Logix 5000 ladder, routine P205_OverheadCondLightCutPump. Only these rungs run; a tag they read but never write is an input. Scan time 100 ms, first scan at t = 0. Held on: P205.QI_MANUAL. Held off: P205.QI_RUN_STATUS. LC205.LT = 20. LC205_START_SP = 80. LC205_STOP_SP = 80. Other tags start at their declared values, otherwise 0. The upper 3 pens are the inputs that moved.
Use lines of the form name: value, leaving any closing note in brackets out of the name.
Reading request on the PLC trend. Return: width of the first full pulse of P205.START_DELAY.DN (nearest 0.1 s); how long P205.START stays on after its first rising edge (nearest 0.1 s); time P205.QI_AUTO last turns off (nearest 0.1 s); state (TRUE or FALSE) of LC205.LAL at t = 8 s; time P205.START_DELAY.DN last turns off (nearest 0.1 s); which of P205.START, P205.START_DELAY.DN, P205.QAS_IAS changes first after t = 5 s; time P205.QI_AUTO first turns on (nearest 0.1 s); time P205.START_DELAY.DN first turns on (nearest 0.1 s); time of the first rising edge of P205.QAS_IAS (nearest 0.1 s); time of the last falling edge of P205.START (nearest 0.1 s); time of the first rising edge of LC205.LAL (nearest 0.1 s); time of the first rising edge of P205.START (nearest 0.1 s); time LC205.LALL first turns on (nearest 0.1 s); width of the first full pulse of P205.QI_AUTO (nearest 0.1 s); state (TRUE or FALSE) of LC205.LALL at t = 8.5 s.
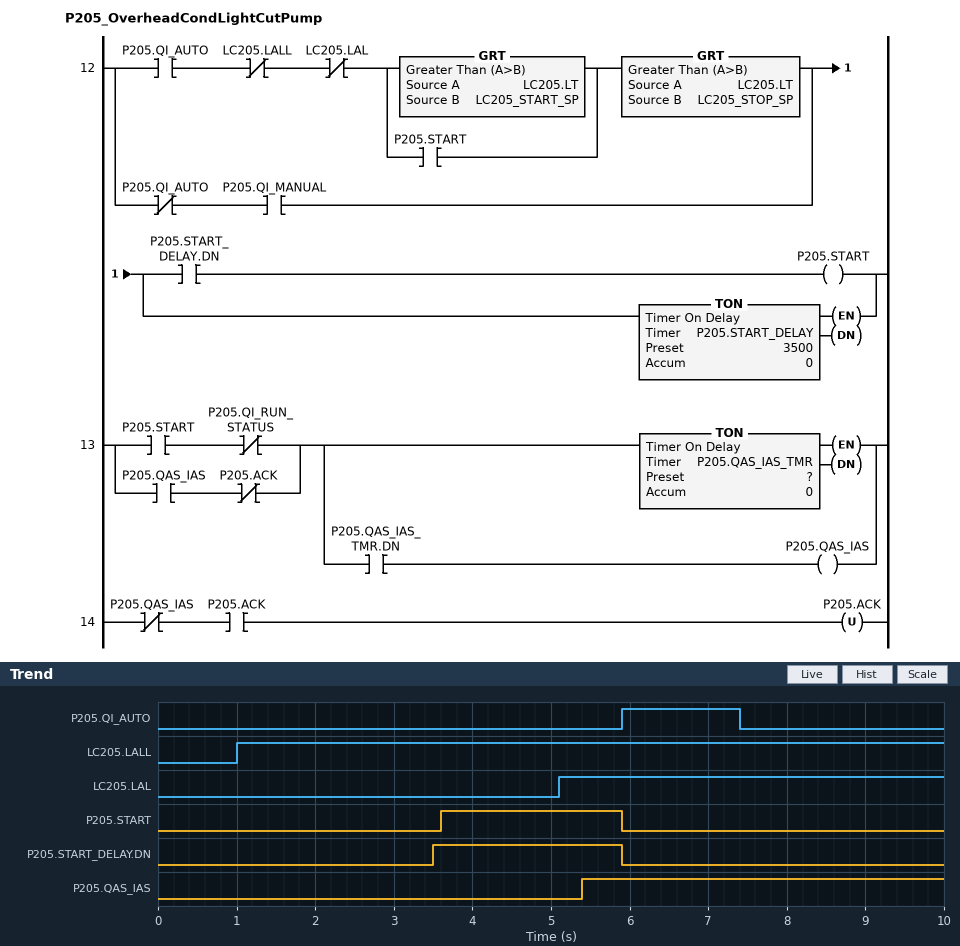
width of the first full pulse of P205.START_DELAY.DN: 2.4 s
how long P205.START stays on after its first rising edge: 2.3 s
time P205.QI_AUTO last turns off: 7.4 s
state (TRUE or FALSE) of LC205.LAL at t = 8 s: TRUE
time P205.START_DELAY.DN last turns off: 5.9 s
which of P205.START, P205.START_DELAY.DN, P205.QAS_IAS changes first after t = 5 s: P205.QAS_IAS
time P205.QI_AUTO first turns on: 5.9 s
time P205.START_DELAY.DN first turns on: 3.5 s
time of the first rising edge of P205.QAS_IAS: 5.4 s
time of the last falling edge of P205.START: 5.9 s
time of the first rising edge of LC205.LAL: 5.1 s
time of the first rising edge of P205.START: 3.6 s
time LC205.LALL first turns on: 1.0 s
width of the first full pulse of P205.QI_AUTO: 1.5 s
state (TRUE or FALSE) of LC205.LALL at t = 8.5 s: TRUE
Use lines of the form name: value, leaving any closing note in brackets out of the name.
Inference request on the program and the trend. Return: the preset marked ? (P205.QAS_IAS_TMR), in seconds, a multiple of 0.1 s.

the preset marked ? (P205.QAS_IAS_TMR), in seconds, a multiple of 0.1 s: 1.8 s
